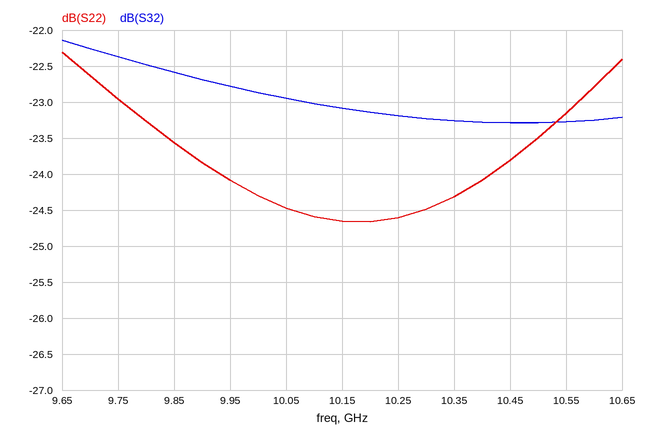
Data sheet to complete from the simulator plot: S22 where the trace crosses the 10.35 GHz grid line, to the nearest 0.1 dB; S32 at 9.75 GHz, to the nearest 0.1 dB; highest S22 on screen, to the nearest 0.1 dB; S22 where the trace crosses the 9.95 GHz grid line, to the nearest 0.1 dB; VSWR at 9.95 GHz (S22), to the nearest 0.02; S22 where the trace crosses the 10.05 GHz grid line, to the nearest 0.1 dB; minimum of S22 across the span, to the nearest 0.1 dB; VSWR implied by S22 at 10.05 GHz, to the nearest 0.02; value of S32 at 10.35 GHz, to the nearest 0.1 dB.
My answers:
-24.3 dB
-22.4 dB
-22.3 dB
-24.1 dB
1.14
-24.5 dB
-24.7 dB
1.12
-23.3 dB
